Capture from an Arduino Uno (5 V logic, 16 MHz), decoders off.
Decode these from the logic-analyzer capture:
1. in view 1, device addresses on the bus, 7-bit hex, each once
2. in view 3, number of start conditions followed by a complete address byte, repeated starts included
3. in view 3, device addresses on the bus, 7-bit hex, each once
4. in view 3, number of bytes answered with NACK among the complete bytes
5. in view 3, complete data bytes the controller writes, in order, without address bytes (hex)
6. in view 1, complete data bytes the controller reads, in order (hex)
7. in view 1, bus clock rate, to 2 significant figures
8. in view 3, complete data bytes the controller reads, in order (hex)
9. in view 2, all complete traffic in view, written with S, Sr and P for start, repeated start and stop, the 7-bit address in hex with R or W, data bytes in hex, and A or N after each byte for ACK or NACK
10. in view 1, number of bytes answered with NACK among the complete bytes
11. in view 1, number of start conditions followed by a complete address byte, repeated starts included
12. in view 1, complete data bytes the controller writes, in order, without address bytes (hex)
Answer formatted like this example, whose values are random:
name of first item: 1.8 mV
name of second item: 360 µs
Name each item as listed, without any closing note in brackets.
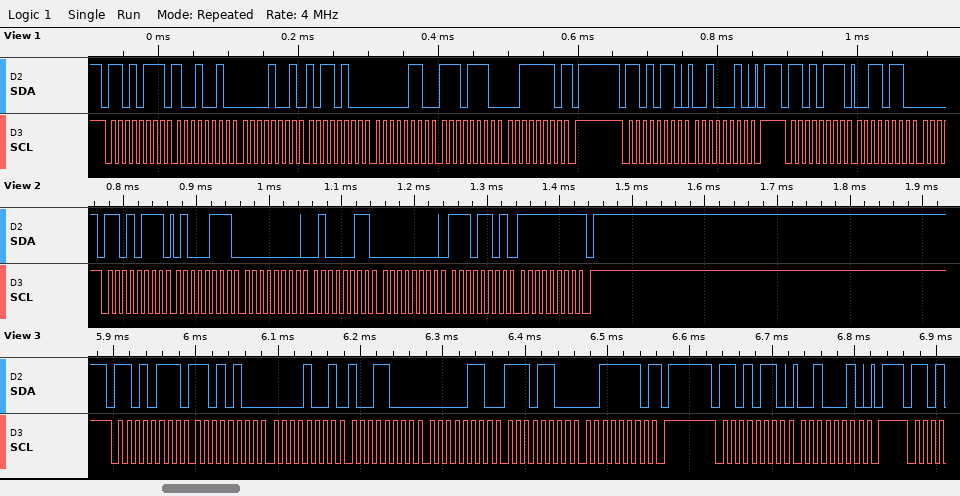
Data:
in view 1, device addresses on the bus, 7-bit hex, each once: 0x6B
in view 3, number of start conditions followed by a complete address byte, repeated starts included: 2
in view 3, device addresses on the bus, 7-bit hex, each once: 0x6B
in view 3, number of bytes answered with NACK among the complete bytes: 1
in view 3, complete data bytes the controller writes, in order, without address bytes: 22
in view 1, complete data bytes the controller reads, in order: 92 09 B4 06 EE 3E 36
in view 1, bus clock rate, to 2 significant figures: 100 kHz
in view 3, complete data bytes the controller reads, in order: D4 09 98 06 EC 3E
in view 2, all complete traffic in view, written with S, Sr and P for start, repeated start and stop, the 7-bit address in hex with R or W, data bytes in hex, and A or N after each byte for ACK or NACK: S 6BR A 47 A 00 A 43 A 00 A ED A FF N P
in view 1, number of bytes answered with NACK among the complete bytes: 1
in view 1, number of start conditions followed by a complete address byte, repeated starts included: 3
in view 1, complete data bytes the controller writes, in order, without address bytes: 22
